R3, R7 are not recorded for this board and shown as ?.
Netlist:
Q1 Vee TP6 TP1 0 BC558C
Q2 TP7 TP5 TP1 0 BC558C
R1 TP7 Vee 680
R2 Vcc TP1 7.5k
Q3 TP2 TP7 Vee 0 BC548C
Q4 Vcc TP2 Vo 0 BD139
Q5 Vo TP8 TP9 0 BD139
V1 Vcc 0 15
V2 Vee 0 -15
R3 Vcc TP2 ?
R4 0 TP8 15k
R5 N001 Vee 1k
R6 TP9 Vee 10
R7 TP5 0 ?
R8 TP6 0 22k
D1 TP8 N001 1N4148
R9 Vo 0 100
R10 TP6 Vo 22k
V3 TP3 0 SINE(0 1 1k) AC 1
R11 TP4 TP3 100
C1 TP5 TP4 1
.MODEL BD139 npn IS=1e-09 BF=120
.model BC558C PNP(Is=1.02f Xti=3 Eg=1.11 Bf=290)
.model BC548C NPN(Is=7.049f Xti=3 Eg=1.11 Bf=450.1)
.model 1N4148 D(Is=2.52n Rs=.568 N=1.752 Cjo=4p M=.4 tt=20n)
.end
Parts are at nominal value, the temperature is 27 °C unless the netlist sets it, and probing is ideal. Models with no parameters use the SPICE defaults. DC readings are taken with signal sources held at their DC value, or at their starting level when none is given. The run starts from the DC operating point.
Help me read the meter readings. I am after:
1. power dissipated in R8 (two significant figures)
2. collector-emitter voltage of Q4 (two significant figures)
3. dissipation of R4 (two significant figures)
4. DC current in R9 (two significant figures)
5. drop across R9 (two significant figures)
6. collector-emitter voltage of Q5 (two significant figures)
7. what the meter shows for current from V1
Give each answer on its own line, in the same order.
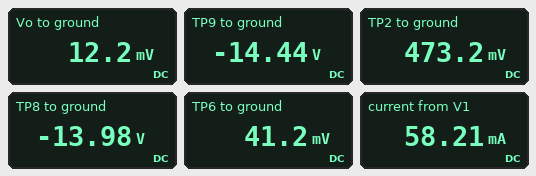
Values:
77 nW
15 V
13 mW
120 µA
12 mV
14 V
58.21 mA
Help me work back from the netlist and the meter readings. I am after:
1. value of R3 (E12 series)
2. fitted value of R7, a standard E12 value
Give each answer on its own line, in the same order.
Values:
12 kΩ
12 kΩ
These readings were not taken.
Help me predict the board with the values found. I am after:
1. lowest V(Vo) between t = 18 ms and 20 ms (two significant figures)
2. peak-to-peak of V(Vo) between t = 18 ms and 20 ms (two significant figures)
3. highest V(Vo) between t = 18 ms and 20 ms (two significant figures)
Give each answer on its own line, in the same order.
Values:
-2.0 V
4.0 V
2.0 V
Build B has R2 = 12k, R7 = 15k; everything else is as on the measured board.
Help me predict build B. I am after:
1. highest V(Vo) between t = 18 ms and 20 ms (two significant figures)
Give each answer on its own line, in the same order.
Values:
2.2 V
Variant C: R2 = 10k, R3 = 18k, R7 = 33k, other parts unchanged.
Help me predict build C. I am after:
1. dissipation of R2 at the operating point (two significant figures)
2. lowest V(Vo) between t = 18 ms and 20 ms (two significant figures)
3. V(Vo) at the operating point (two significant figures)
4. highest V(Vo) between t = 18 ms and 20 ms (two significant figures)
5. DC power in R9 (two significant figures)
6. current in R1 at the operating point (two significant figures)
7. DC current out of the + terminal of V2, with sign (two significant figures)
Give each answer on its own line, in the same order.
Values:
20 mW
-1.8 V
210 mV
2.2 V
440 µW
930 µA
-58 mA
